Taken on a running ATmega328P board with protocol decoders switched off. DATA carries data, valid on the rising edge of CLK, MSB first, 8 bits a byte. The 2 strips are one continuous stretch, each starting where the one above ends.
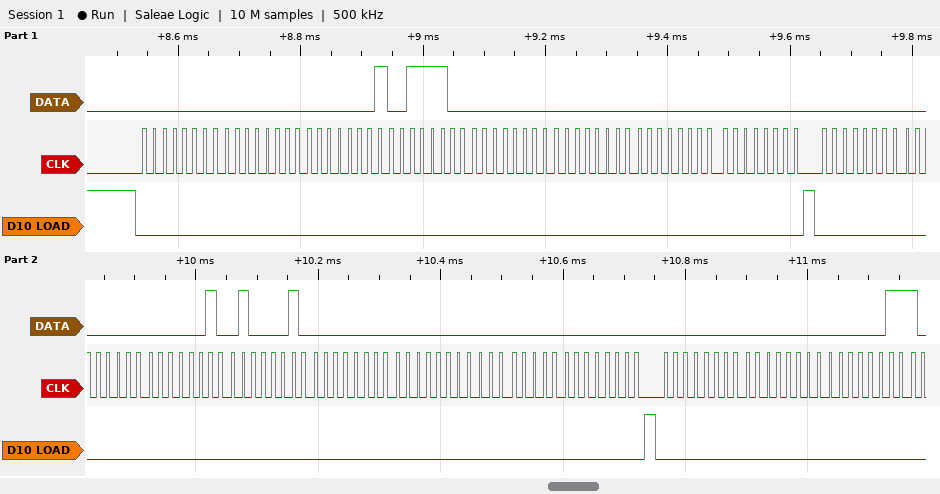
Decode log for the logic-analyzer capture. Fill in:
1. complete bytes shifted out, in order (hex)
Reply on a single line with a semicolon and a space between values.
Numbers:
00 00 01 3C 00 00 00 00 00 00 02 42 00 00 00 00 00 00 03
